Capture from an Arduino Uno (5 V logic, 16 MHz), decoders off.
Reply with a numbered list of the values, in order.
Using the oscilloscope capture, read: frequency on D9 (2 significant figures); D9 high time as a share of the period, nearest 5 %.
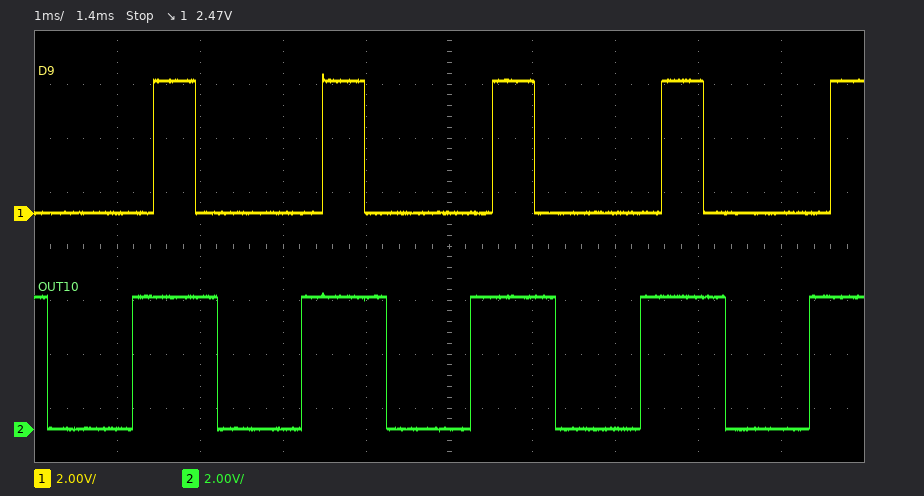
1. 490 Hz
2. 25 %
